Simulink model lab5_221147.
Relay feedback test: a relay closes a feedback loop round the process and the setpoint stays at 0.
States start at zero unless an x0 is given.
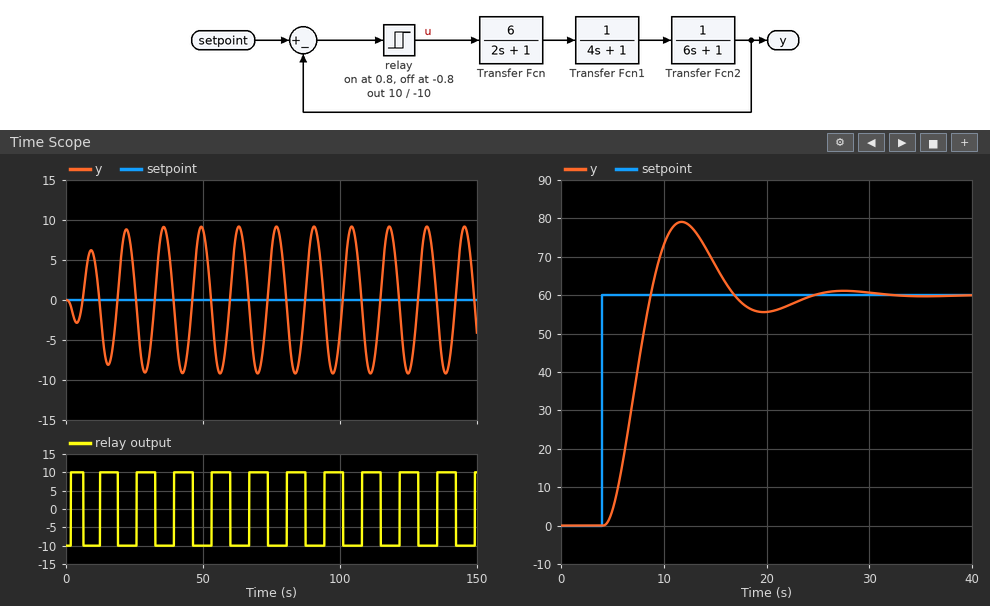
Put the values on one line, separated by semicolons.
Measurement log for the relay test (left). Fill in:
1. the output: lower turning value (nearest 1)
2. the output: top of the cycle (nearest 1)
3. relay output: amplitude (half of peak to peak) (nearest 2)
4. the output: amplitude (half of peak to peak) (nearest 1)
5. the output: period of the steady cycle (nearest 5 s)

-9; 9; 10; 9; 15 s
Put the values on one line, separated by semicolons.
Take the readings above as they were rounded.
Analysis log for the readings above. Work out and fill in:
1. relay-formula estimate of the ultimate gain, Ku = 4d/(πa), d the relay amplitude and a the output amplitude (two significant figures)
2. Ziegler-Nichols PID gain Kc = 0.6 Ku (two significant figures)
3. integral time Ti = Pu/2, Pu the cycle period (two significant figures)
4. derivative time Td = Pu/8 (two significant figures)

1.4; 0.84; 7.5 s; 1.9 s
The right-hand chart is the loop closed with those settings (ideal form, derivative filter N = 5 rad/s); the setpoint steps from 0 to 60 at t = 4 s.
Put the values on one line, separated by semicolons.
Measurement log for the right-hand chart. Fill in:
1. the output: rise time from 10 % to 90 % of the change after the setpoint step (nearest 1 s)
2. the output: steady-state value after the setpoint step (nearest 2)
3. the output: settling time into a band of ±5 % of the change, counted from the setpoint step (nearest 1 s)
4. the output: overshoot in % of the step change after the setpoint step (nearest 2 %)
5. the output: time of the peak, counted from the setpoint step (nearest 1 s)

3 s; 60; 18 s; 32 %; 8 s
